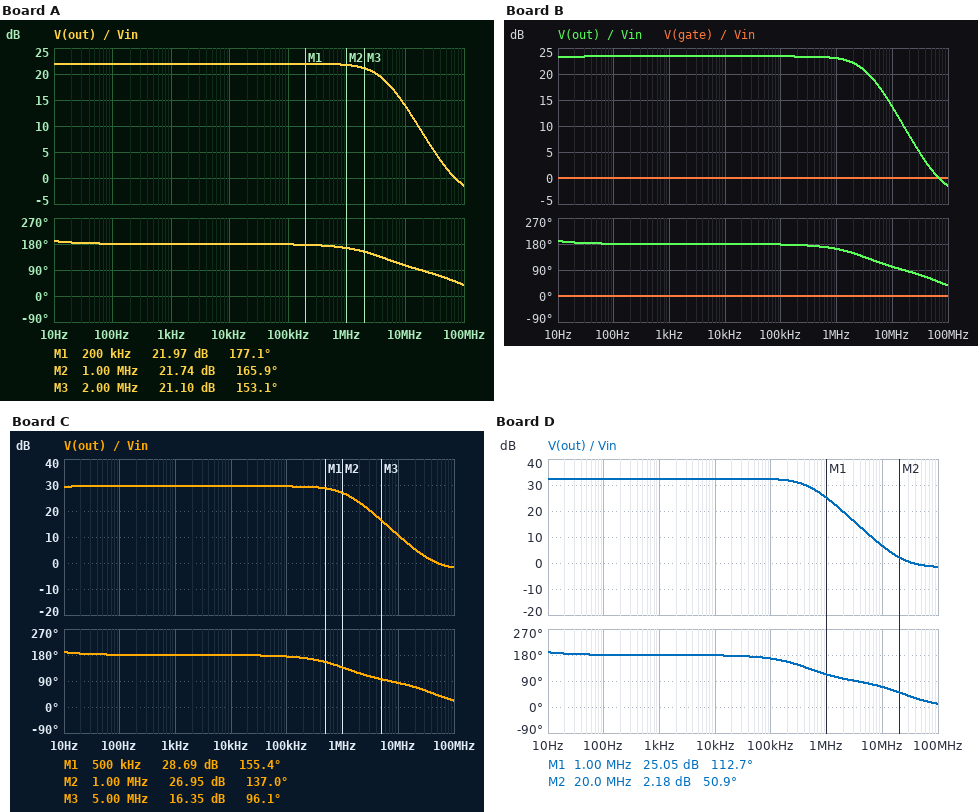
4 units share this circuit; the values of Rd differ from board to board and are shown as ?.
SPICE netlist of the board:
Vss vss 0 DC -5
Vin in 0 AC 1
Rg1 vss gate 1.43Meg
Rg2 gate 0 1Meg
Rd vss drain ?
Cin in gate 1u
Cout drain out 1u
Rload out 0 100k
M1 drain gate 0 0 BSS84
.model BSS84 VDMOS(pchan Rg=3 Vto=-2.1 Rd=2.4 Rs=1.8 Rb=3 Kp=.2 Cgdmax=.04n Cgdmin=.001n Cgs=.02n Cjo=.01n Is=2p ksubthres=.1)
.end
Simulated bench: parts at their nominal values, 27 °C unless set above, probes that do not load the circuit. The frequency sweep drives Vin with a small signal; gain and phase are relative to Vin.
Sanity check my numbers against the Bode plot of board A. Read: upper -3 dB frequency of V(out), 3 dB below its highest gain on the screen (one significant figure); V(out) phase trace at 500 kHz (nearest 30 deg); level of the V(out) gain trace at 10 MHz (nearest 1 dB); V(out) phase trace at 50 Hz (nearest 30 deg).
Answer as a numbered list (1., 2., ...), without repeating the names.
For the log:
1. 4 MHz
2. 180 deg
3. 14 dB
4. 180 deg
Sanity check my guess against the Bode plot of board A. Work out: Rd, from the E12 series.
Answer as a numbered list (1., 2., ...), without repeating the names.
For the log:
1. 3.3 kΩ
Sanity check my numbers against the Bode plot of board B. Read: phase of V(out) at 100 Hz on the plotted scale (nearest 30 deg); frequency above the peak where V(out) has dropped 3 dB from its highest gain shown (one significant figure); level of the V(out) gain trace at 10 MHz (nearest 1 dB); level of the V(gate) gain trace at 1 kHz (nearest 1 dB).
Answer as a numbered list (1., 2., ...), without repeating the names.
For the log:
1. 180 deg
2. 3 MHz
3. 14 dB
4. 0 dB
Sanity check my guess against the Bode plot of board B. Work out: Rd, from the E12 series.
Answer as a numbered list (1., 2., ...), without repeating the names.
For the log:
1. 3.9 kΩ
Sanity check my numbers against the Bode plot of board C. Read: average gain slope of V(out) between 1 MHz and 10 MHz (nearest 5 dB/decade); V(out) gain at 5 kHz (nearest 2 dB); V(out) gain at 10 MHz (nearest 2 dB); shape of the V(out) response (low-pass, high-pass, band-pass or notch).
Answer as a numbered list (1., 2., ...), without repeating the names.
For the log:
1. -15 dB/decade
2. 30 dB
3. 10 dB
4. low-pass
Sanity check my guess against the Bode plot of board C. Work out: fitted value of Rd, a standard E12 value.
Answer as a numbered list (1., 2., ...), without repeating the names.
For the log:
1. 8.2 kΩ
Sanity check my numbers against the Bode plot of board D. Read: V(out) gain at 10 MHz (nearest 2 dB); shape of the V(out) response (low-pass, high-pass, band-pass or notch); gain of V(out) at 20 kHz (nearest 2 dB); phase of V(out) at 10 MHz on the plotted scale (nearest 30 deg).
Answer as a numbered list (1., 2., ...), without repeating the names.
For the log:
1. 6 dB
2. low-pass
3. 32 dB
4. 60 deg
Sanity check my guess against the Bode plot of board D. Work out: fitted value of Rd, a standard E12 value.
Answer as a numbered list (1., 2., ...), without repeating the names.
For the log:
1. 12 kΩ
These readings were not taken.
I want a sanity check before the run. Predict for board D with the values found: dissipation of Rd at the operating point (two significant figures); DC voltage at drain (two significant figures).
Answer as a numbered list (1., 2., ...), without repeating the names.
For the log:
1. 760 µW
2. -2.0 V
